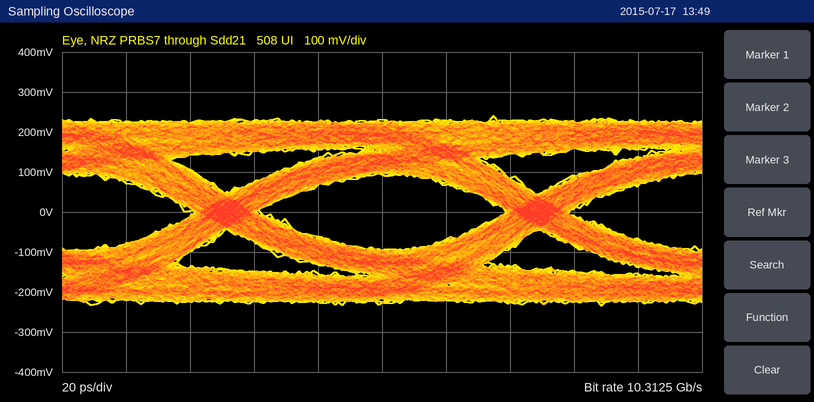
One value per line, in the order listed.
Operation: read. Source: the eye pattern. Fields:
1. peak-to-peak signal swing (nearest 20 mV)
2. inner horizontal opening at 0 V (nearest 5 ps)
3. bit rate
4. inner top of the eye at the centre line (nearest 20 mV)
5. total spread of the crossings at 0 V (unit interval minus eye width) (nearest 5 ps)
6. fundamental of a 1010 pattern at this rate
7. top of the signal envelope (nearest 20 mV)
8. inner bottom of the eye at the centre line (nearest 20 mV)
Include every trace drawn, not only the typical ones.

480 mV
75 ps
10.3125 Gb/s
100 mV
20 ps
5.15625 GHz
240 mV
-100 mV
